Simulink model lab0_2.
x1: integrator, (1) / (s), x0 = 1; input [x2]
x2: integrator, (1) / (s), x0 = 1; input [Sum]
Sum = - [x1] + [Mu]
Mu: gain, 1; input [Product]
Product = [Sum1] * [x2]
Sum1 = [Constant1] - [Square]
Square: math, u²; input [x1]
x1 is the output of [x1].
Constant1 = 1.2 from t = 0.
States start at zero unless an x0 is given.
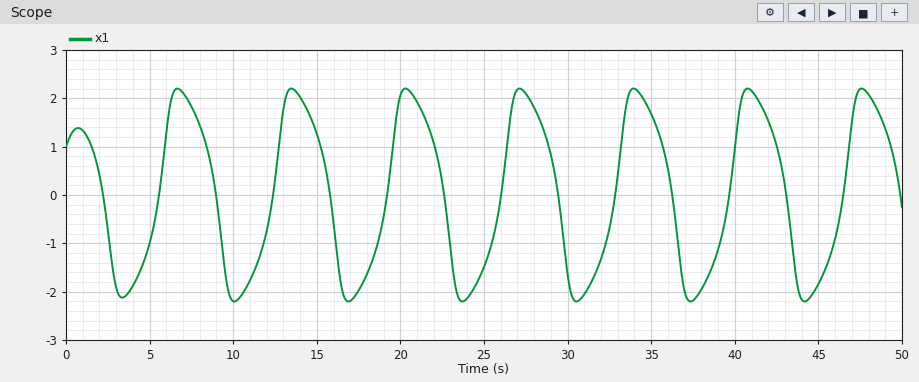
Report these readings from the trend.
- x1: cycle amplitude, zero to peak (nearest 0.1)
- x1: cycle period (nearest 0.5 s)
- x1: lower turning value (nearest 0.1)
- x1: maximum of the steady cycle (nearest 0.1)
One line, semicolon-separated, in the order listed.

2.2; 7.0 s; -2.2; 2.2
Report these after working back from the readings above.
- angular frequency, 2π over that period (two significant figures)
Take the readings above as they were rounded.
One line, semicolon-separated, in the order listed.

0.90 rad/s
